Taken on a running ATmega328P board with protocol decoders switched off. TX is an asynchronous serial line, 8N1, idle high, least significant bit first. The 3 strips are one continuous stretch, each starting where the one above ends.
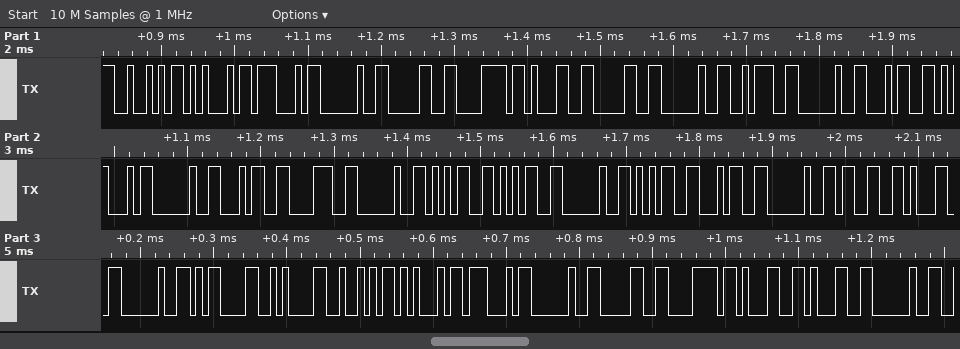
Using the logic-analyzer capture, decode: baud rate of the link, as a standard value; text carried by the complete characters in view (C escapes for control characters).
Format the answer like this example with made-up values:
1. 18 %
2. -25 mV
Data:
1. 115200 baud
2. "REG 0x10 : 4E 48 55 54 31 \r\nREG 0x11 "
